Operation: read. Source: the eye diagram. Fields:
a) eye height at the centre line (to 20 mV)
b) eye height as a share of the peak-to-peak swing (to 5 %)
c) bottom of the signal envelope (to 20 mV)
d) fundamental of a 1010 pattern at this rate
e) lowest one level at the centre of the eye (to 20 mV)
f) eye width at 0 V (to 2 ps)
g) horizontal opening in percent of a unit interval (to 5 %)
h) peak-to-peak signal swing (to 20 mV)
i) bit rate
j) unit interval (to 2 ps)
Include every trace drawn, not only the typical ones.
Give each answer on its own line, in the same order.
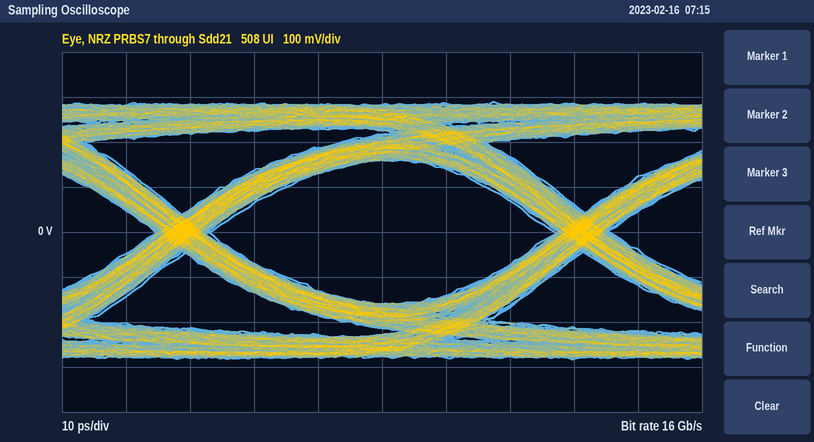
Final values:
320 mV
55 %
-280 mV
8 GHz
160 mV
54 ps
85 %
580 mV
16 Gb/s
62 ps
